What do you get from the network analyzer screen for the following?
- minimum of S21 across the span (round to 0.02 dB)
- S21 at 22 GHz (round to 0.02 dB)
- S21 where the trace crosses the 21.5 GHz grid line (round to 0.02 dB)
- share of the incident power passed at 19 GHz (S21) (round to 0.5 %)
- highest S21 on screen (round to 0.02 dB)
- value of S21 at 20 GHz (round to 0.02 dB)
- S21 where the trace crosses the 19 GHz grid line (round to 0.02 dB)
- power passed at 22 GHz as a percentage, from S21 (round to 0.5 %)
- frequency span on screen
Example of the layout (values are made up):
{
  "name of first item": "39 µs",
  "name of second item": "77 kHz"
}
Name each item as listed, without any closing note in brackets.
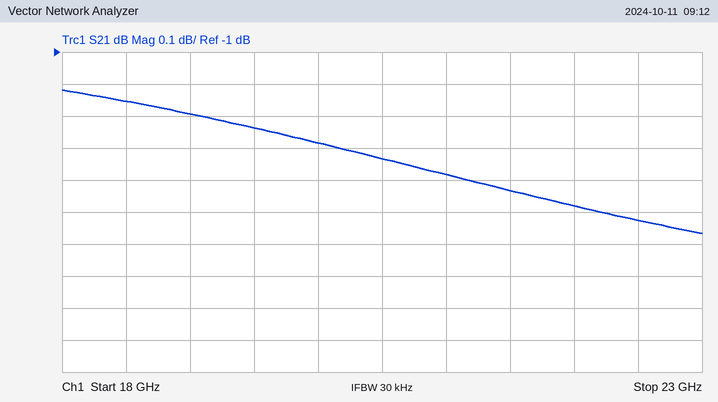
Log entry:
{
  "minimum of S21 across the span": "-1.56 dB",
  "S21 at 22 GHz": "-1.48 dB",
  "S21 where the trace crosses the 21.5 GHz grid line": "-1.44 dB",
  "share of the incident power passed at 19 GHz (S21)": "76.0 %",
  "highest S21 on screen": "-1.12 dB",
  "value of S21 at 20 GHz": "-1.28 dB",
  "S21 where the trace crosses the 19 GHz grid line": "-1.20 dB",
  "power passed at 22 GHz as a percentage, from S21": "71.0 %",
  "frequency span on screen": "5 GHz"
}
